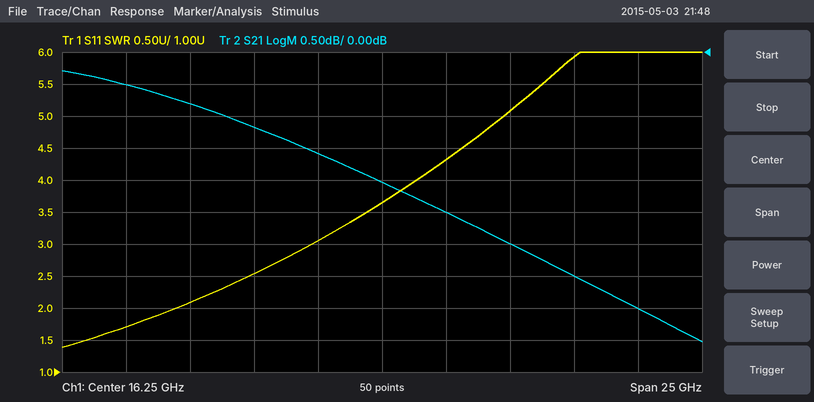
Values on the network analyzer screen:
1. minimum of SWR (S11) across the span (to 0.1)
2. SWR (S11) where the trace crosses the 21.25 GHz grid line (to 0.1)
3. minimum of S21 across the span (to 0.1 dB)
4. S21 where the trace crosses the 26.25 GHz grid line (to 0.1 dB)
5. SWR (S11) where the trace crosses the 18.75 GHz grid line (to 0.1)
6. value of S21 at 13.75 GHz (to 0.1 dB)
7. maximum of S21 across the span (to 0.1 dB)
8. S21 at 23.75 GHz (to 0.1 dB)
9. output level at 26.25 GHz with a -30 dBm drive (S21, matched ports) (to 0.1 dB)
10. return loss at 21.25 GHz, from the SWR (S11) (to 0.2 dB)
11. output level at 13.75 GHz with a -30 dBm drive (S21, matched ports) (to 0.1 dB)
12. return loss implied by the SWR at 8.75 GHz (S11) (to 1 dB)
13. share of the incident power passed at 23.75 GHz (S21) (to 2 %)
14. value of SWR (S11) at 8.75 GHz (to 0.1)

1.4
5.1
-4.5 dB
-4.0 dB
4.3
-1.6 dB
-0.3 dB
-3.5 dB
-34.0 dBm
3.4 dB
-31.6 dBm
9 dB
44 %
2.1
